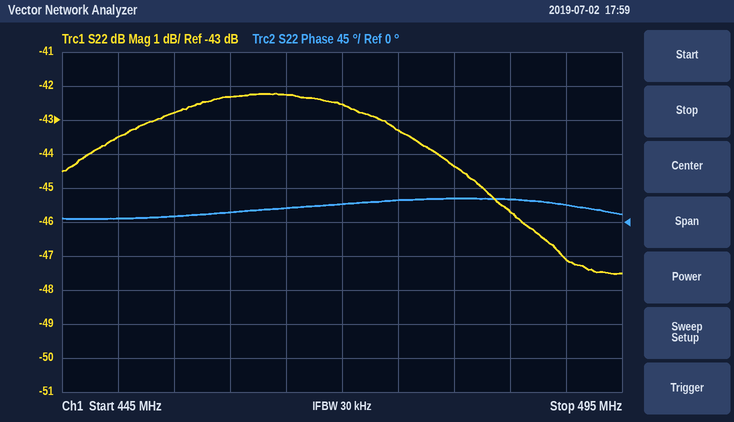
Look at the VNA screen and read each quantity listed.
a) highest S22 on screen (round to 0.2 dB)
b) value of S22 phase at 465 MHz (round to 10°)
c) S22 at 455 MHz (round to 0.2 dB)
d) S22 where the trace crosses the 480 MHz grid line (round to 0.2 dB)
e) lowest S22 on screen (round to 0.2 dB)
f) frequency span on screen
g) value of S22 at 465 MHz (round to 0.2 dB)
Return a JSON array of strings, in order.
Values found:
["-42.2 dB", "20°", "-42.8 dB", "-44.4 dB", "-47.6 dB", "50 MHz", "-42.2 dB"]
